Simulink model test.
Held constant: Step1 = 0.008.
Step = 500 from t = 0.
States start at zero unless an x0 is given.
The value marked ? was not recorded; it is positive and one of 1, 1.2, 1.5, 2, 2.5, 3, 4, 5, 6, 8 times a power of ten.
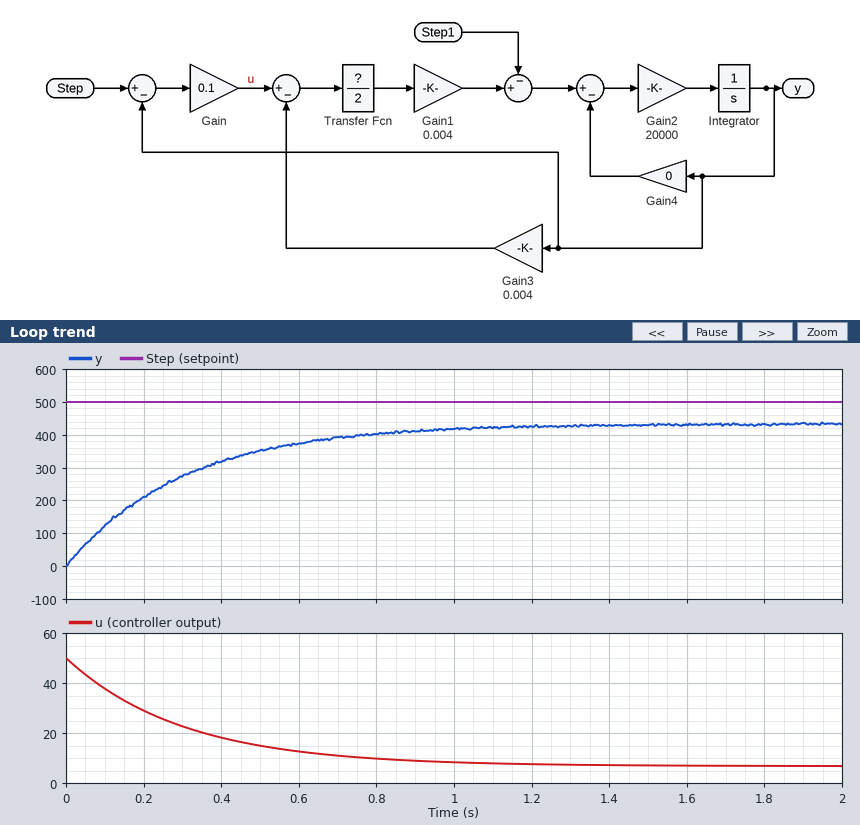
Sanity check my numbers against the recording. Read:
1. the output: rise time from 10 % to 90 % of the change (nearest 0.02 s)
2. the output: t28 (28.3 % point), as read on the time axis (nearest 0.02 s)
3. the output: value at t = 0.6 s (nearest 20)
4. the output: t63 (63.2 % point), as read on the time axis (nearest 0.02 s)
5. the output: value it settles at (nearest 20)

0.66 s
0.10 s
380
0.30 s
440
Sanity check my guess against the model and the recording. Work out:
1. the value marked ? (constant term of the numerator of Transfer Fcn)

0.8
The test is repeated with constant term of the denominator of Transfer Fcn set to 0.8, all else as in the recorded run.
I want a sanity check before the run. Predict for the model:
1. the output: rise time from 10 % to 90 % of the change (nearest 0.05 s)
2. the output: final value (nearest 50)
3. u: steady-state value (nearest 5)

0.25 s
450
5
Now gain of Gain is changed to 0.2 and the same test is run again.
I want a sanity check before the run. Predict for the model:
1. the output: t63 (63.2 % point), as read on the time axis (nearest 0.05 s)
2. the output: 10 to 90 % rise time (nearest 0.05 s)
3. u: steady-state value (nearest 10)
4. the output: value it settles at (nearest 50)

0.15 s
0.35 s
10
450
